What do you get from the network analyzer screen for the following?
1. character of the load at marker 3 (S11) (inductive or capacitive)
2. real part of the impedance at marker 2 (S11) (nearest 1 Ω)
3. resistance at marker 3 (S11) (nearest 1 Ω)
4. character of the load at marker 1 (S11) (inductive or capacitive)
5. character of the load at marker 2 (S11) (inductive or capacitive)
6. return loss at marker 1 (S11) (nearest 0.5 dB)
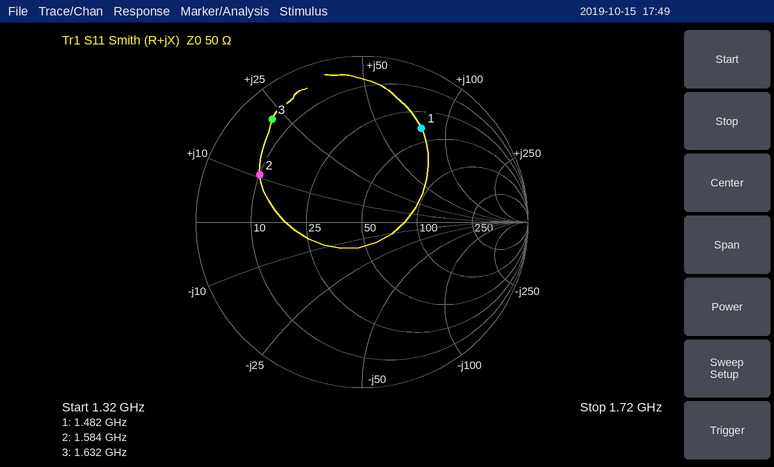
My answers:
inductive
10 Ω
6 Ω
inductive
inductive
3.5 dB
